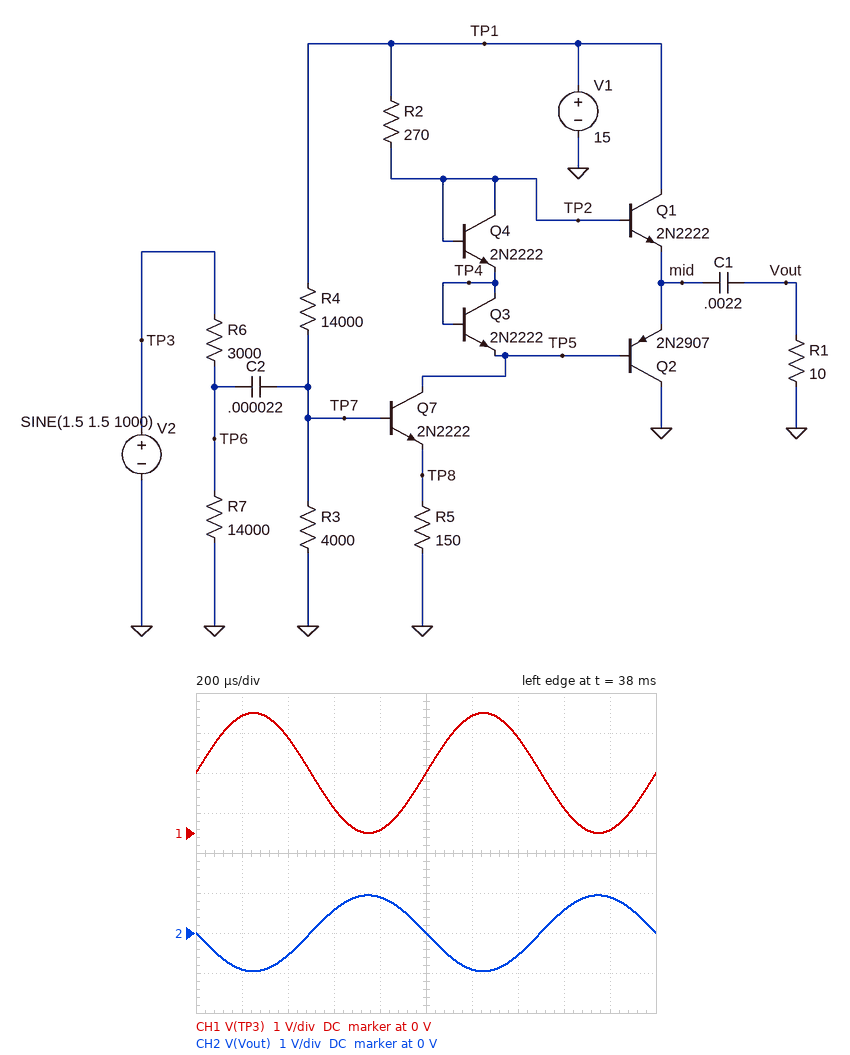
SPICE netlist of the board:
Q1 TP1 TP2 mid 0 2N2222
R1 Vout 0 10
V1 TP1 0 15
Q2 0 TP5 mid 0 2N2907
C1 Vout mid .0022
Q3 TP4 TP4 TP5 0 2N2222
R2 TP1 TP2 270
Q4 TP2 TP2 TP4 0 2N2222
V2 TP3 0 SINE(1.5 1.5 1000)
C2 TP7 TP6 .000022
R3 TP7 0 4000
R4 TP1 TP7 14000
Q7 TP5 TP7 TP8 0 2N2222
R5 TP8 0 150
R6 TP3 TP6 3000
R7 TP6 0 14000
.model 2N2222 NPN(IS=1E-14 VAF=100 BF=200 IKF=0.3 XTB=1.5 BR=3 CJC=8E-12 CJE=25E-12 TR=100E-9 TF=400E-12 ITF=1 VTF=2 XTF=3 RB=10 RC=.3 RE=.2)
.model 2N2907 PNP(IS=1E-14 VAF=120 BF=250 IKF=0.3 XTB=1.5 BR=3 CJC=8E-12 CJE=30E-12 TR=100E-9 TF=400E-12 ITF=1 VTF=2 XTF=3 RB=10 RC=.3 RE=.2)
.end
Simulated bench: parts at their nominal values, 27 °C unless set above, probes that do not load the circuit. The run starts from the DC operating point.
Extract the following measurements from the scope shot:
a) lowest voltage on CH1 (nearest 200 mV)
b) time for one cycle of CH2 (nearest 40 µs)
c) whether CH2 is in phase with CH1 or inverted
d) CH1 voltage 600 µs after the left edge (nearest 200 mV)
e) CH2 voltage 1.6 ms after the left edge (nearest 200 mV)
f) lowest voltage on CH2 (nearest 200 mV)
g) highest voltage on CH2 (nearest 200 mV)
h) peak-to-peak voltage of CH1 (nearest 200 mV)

0 V
1.00 ms
inverted
600 mV
600 mV
-1.0 V
1.0 V
3.0 V
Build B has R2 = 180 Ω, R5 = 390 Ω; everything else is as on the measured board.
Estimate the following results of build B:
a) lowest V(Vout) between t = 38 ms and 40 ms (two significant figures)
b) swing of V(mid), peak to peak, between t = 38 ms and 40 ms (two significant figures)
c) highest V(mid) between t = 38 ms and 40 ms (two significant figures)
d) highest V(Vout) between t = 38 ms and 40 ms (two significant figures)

-250 mV
500 mV
13 V
250 mV
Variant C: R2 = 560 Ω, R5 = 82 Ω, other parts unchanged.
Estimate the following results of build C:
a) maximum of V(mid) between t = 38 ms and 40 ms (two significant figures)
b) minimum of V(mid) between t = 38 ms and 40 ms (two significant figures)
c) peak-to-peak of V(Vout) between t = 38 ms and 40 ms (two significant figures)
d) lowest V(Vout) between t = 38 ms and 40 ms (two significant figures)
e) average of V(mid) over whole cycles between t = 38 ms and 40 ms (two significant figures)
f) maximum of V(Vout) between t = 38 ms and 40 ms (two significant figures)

4.7 V
2.6 V
2.1 V
-440 mV
3.2 V
1.7 V
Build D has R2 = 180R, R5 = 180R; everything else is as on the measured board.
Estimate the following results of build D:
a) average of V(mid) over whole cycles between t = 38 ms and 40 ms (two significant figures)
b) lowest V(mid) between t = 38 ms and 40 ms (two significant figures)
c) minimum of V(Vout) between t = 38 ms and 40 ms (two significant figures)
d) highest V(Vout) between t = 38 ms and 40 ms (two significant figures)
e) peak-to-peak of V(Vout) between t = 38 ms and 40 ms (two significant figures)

12 V
11 V
-560 mV
550 mV
1.1 V
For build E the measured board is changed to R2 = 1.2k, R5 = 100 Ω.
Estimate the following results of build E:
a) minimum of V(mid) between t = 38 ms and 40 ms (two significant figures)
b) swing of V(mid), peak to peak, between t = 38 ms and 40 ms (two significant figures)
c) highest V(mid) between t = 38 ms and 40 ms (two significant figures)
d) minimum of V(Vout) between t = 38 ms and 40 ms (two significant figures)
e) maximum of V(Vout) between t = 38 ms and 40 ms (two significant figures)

1.9 V
260 mV
2.1 V
-26 mV
230 mV
